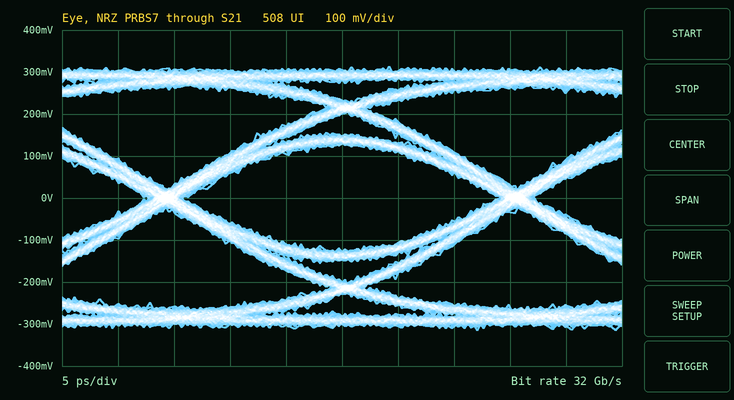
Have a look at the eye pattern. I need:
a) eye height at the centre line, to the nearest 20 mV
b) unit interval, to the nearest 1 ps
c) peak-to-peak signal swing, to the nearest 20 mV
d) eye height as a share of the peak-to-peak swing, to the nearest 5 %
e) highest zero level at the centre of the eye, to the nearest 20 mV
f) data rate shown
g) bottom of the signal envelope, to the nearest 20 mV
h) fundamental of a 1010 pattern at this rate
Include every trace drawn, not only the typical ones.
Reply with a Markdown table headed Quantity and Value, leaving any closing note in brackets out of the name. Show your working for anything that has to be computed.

| Quantity | Value |
|---|---|
| eye height at the centre line, to the nearest 20 mV | 260 mV |
| unit interval, to the nearest 1 ps | 31 ps |
| peak-to-peak signal swing, to the nearest 20 mV | 620 mV |
| eye height as a share of the peak-to-peak swing, to the nearest 5 % | 260 mV / 620 mV ≈ 41.9 %, so 40 % to the nearest 5 % |
| highest zero level at the centre of the eye, to the nearest 20 mV | -120 mV |
| data rate shown | 32 Gb/s |
| bottom of the signal envelope, to the nearest 20 mV | -320 mV |
| fundamental of a 1010 pattern at this rate | 16 GHz |
